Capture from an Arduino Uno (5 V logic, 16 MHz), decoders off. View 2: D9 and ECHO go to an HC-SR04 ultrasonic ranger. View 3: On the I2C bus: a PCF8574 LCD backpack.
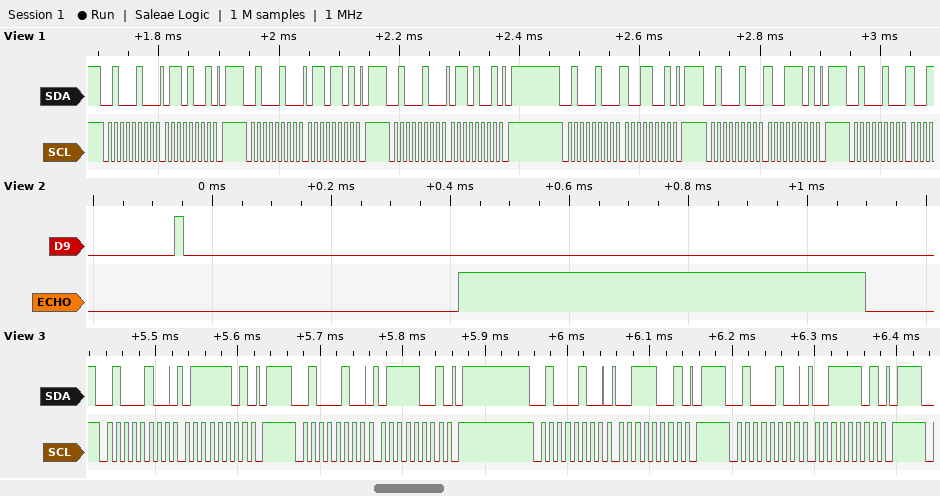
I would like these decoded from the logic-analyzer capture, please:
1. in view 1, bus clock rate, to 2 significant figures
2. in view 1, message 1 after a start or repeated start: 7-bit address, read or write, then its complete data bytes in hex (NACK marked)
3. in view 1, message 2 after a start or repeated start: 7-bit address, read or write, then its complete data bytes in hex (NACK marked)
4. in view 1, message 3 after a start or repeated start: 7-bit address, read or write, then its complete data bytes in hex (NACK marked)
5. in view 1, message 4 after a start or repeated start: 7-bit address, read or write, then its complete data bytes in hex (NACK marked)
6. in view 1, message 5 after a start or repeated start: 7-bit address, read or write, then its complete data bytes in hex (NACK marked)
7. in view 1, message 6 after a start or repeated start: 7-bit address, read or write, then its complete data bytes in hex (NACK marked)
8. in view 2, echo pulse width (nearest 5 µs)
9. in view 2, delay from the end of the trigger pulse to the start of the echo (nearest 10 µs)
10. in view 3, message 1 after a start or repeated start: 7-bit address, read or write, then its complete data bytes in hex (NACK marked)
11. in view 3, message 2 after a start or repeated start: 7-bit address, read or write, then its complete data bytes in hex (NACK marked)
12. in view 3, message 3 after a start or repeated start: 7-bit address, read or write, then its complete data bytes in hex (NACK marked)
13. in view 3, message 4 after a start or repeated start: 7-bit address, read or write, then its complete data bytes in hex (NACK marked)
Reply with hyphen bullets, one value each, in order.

- 100 kHz
- 0x22 write: 69
- 0x22 write: 6D
- 0x22 write: 69
- 0x22 write: 99
- 0x22 write: 9D
- 0x22 write
- 685 µs
- 460 µs
- 0x22 write: 7D
- 0x22 write: 79
- 0x22 write: 39
- 0x22 write: 3D
